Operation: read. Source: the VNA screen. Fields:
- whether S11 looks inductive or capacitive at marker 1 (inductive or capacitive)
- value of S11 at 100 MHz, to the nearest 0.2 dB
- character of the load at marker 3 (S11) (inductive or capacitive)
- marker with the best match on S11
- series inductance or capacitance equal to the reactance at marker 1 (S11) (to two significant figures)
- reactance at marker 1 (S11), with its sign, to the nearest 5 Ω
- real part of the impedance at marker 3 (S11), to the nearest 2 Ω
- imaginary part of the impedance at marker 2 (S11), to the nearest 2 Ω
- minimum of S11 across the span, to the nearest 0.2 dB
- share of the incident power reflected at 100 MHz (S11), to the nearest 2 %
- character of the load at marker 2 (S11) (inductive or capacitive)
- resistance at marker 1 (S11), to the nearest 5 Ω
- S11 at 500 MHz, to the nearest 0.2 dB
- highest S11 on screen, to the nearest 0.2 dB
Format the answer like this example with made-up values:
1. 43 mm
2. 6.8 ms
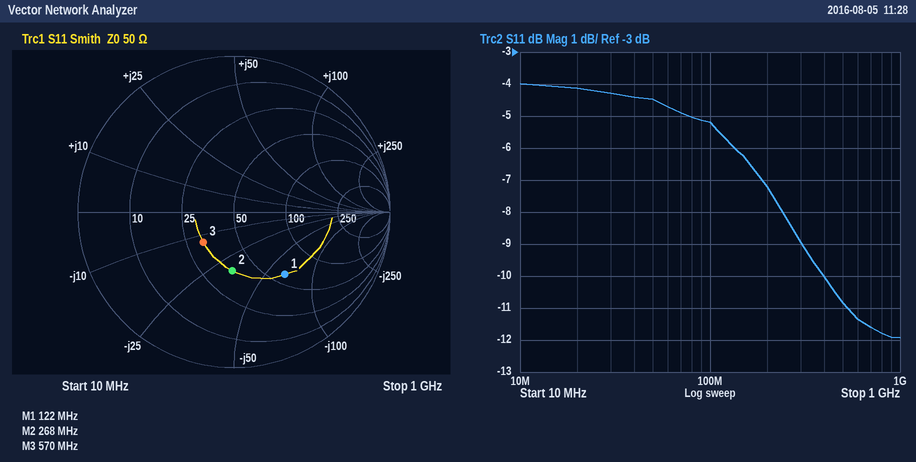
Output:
1. capacitive
2. -5.2 dB
3. capacitive
4. marker 3
5. 20 pF
6. -65 Ω
7. 32 Ω
8. -32 Ω
9. -12.0 dB
10. 30 %
11. capacitive
12. 60 Ω
13. -10.8 dB
14. -4.0 dB
